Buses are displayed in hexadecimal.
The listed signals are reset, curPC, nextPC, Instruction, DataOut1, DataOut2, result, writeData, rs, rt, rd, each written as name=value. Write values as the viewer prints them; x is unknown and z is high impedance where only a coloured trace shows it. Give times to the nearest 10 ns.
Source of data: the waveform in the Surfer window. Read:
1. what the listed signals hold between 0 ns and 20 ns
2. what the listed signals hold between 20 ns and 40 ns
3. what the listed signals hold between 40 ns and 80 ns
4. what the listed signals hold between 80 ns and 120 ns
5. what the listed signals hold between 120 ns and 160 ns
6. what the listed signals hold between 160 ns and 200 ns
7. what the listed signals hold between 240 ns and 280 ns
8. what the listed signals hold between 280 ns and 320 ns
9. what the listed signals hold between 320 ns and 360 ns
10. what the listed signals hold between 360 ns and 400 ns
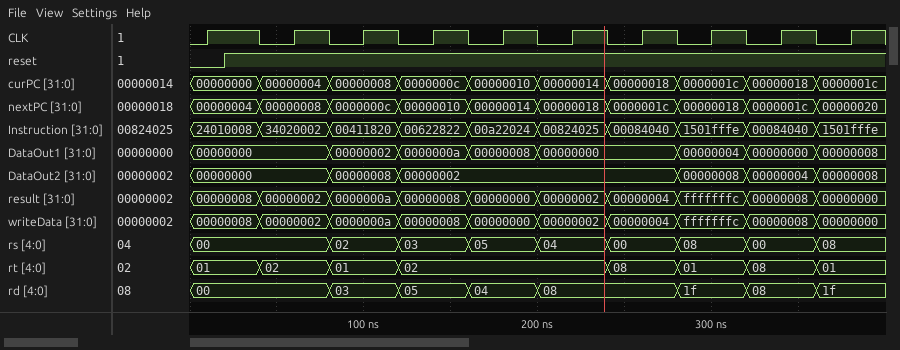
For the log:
reset=0, curPC=00000000, nextPC=00000004, Instruction=24010008, DataOut1=00000000, DataOut2=00000000, result=00000008, writeData=00000008, rs=00, rt=01, rd=00
reset=1, curPC=00000000, nextPC=00000004, Instruction=24010008, DataOut1=00000000, DataOut2=00000000, result=00000008, writeData=00000008, rs=00, rt=01, rd=00
reset=1, curPC=00000004, nextPC=00000008, Instruction=34020002, DataOut1=00000000, DataOut2=00000000, result=00000002, writeData=00000002, rs=00, rt=02, rd=00
reset=1, curPC=00000008, nextPC=0000000c, Instruction=00411820, DataOut1=00000002, DataOut2=00000008, result=0000000a, writeData=0000000a, rs=02, rt=01, rd=03
reset=1, curPC=0000000c, nextPC=00000010, Instruction=00622822, DataOut1=0000000a, DataOut2=00000002, result=00000008, writeData=00000008, rs=03, rt=02, rd=05
reset=1, curPC=00000010, nextPC=00000014, Instruction=00a22024, DataOut1=00000008, DataOut2=00000002, result=00000000, writeData=00000000, rs=05, rt=02, rd=04
reset=1, curPC=00000018, nextPC=0000001c, Instruction=00084040, DataOut1=00000000, DataOut2=00000002, result=00000004, writeData=00000004, rs=00, rt=08, rd=08
reset=1, curPC=0000001c, nextPC=00000018, Instruction=1501fffe, DataOut1=00000004, DataOut2=00000008, result=fffffffc, writeData=fffffffc, rs=08, rt=01, rd=1f
reset=1, curPC=00000018, nextPC=0000001c, Instruction=00084040, DataOut1=00000000, DataOut2=00000004, result=00000008, writeData=00000008, rs=00, rt=08, rd=08
reset=1, curPC=0000001c, nextPC=00000020, Instruction=1501fffe, DataOut1=00000008, DataOut2=00000008, result=00000000, writeData=00000000, rs=08, rt=01, rd=1f
